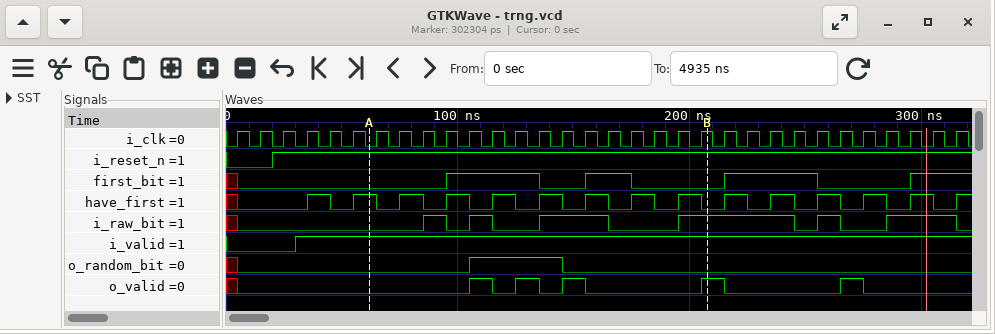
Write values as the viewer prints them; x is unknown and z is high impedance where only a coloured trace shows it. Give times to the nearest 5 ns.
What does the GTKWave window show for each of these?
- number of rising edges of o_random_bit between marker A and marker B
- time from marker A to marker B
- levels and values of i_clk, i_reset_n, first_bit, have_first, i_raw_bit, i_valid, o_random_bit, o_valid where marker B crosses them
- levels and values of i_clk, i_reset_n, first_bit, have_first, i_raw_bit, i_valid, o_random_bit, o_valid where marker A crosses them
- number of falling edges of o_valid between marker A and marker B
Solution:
1
145 ns
i_clk=1, i_reset_n=1, first_bit=0, have_first=0, i_raw_bit=1, i_valid=1, o_random_bit=0, o_valid=1
i_clk=0, i_reset_n=1, first_bit=0, have_first=1, i_raw_bit=0, i_valid=1, o_random_bit=0, o_valid=0
3
